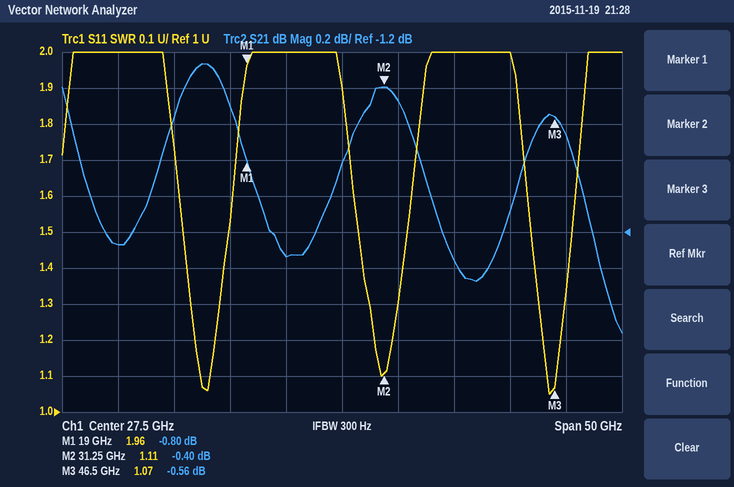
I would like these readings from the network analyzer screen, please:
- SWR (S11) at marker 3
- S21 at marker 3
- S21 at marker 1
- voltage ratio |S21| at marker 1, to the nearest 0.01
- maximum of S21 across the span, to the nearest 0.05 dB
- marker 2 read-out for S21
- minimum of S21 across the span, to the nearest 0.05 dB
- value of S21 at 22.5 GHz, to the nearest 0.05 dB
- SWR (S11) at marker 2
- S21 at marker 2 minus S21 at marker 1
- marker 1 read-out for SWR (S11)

1.07
-0.56 dB
-0.80 dB
0.91
-0.25 dB
-0.40 dB
-1.75 dB
-1.35 dB
1.11
0.40 dB
1.96
